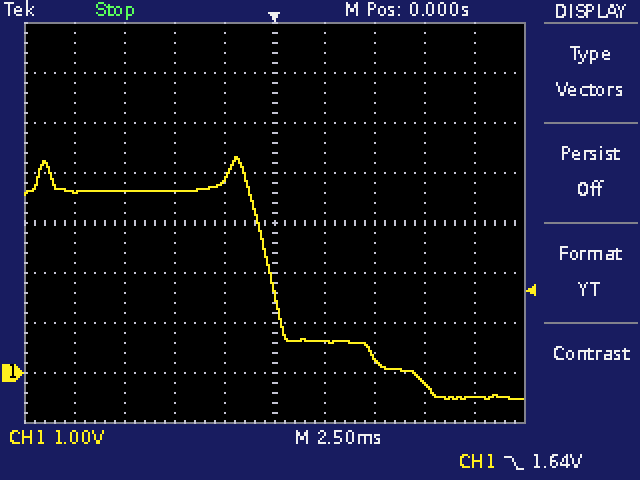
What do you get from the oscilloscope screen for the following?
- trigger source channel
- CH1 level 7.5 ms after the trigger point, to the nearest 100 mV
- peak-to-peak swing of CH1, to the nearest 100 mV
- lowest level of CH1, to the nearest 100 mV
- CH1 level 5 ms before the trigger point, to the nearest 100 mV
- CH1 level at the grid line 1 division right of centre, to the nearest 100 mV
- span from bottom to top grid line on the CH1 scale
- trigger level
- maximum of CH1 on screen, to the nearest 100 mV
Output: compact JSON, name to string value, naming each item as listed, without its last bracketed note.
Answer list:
{"trigger source channel": "CH1", "CH1 level 7.5 ms after the trigger point, to the nearest 100 mV": "-200 mV", "peak-to-peak swing of CH1, to the nearest 100 mV": "4.8 V", "lowest level of CH1, to the nearest 100 mV": "-500 mV", "CH1 level 5 ms before the trigger point, to the nearest 100 mV": "3.6 V", "CH1 level at the grid line 1 division right of centre, to the nearest 100 mV": "600 mV", "span from bottom to top grid line on the CH1 scale": "8 V", "trigger level": "1.64 V", "maximum of CH1 on screen, to the nearest 100 mV": "4.3 V"}
